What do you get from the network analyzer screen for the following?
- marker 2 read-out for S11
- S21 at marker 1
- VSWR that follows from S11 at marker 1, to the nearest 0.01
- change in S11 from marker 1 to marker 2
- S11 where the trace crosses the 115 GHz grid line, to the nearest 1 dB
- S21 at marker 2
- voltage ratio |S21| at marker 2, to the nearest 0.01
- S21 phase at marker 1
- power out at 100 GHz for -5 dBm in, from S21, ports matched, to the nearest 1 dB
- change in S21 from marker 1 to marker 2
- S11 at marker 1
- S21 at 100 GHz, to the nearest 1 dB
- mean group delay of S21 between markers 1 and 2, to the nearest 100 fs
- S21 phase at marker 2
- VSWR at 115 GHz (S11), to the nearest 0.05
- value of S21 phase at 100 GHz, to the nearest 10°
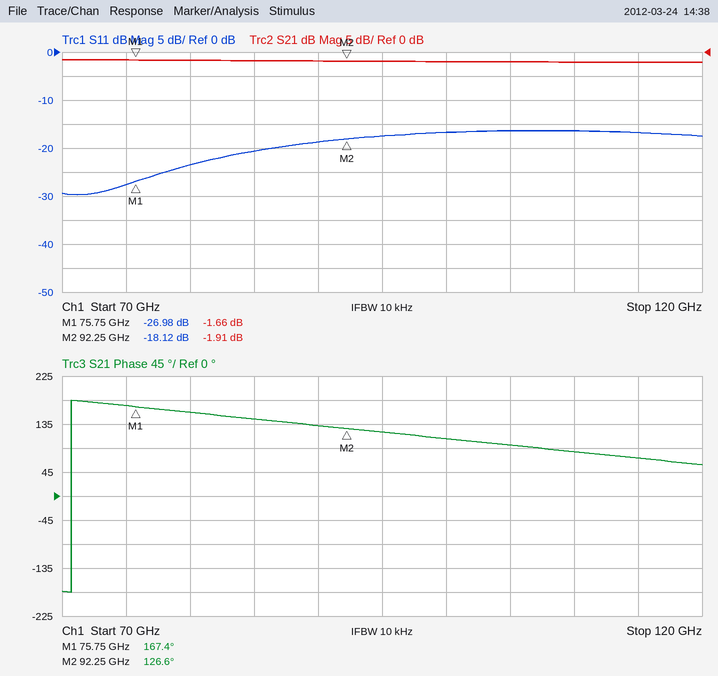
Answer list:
-18.12 dB
-1.66 dB
1.09
8.86 dB
-17 dB
-1.91 dB
0.80
167.4°
-7 dBm
-0.25 dB
-26.98 dB
-2 dB
6.9 ps
126.6°
1.35
110°
